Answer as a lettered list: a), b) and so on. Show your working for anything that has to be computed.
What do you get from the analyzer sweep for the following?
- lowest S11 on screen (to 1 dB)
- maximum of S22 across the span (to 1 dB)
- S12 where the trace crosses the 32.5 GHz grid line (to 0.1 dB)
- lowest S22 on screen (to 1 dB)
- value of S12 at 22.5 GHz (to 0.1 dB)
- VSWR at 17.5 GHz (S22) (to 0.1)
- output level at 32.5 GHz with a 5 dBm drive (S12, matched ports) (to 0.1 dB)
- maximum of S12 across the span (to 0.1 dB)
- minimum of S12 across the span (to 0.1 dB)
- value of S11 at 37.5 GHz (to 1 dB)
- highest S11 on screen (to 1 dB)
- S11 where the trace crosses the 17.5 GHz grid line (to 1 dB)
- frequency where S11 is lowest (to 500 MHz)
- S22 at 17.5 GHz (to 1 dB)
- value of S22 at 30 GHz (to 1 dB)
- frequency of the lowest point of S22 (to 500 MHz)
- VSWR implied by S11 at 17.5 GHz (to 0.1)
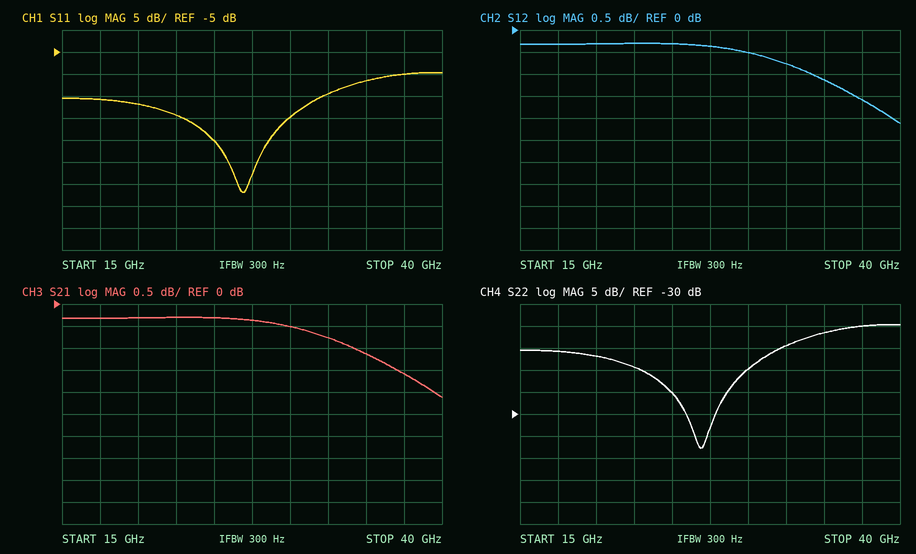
a) -37 dB
b) -10 dB
c) -0.8 dB
d) -38 dB
e) -0.3 dB
f) |Γ| = 10^(-16/20) = 0.1585; VSWR = (1 + 0.1585)/(1 − 0.1585) ≈ 1.4
g) 5 dBm + (-0.8 dB) = 4.2 dBm
h) -0.3 dB
i) -2.1 dB
j) -10 dB
k) -10 dB
l) -16 dB
m) 27.0 GHz
n) -16 dB
o) -20 dB
p) 27.0 GHz
q) |Γ| = 10^(-16/20) = 0.1585; VSWR = (1 + 0.1585)/(1 − 0.1585) ≈ 1.4
